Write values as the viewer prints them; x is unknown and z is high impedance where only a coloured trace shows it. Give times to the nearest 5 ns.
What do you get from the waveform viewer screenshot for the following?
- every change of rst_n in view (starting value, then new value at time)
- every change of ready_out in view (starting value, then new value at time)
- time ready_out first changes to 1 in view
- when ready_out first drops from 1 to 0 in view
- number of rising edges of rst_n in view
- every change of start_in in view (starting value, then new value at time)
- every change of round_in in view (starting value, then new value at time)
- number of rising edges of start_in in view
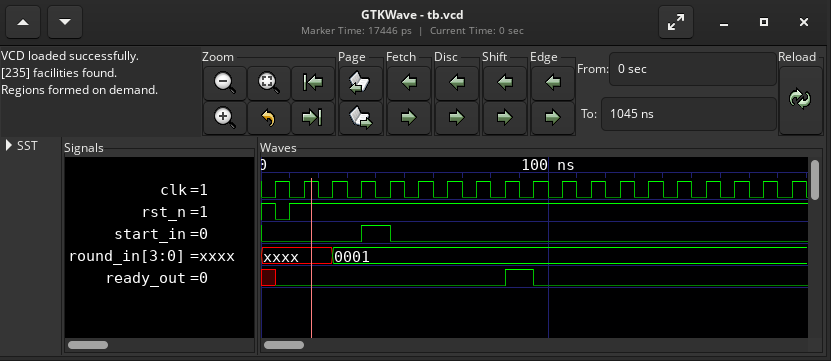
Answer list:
1, 0 at 5 ns, 1 at 10 ns
x, 0 at 5 ns, 1 at 85 ns, 0 at 95 ns
85 ns
95 ns
1
0, 1 at 35 ns, 0 at 45 ns
xxxx, 0001 at 25 ns
1
